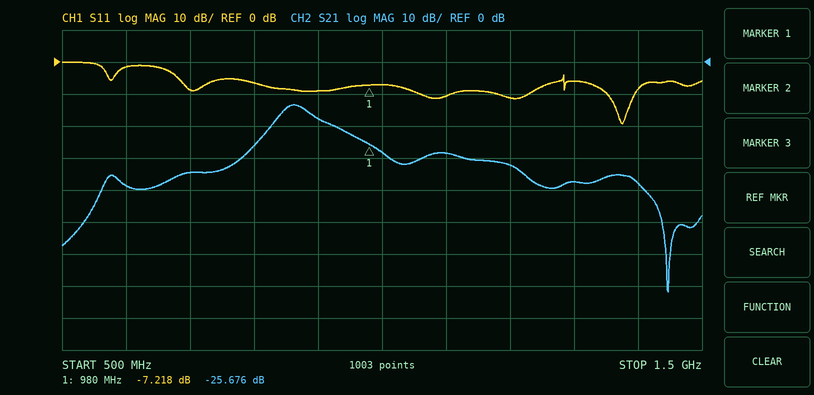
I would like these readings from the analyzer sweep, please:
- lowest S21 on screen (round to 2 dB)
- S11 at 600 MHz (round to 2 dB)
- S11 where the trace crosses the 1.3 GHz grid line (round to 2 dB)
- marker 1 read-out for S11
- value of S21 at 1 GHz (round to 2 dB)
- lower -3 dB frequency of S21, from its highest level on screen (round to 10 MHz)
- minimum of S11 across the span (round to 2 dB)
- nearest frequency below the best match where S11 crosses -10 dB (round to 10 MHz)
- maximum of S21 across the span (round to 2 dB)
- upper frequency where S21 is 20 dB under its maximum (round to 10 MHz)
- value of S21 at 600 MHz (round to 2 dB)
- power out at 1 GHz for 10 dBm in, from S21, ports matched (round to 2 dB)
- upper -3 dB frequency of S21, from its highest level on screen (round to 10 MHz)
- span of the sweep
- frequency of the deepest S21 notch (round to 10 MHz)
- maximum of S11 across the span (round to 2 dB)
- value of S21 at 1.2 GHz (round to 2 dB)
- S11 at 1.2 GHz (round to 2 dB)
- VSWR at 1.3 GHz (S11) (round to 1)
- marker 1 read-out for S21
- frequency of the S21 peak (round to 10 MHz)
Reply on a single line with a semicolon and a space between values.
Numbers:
-72 dB; -2 dB; -6 dB; -7.218 dB; -28 dB; 840 MHz; -20 dB; 1.35 GHz; -14 dB; 1.21 GHz; -38 dB; -18 dBm; 890 MHz; 1 GHz; 1.45 GHz; 0 dB; -32 dB; -12 dB; 3; -25.676 dB; 860 MHz
